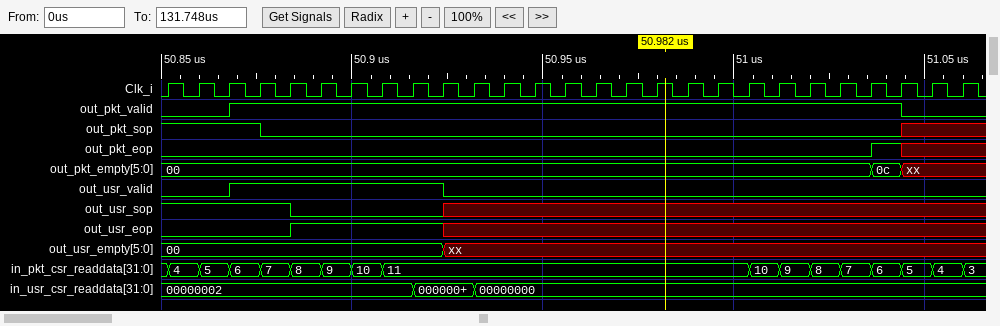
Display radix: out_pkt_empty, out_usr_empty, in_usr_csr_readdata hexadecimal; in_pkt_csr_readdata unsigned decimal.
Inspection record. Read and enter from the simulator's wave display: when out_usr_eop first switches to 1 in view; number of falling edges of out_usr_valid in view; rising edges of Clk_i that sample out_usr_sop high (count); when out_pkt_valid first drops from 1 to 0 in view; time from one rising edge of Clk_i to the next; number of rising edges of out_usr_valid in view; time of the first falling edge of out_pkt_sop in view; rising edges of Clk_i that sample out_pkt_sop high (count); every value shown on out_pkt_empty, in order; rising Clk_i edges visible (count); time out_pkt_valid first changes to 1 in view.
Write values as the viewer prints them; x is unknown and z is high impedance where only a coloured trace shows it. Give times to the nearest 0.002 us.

50.884 us
1
5
51.044 us
0.008 us
1
50.876 us
4
00, 0c, xx
27
50.868 us
